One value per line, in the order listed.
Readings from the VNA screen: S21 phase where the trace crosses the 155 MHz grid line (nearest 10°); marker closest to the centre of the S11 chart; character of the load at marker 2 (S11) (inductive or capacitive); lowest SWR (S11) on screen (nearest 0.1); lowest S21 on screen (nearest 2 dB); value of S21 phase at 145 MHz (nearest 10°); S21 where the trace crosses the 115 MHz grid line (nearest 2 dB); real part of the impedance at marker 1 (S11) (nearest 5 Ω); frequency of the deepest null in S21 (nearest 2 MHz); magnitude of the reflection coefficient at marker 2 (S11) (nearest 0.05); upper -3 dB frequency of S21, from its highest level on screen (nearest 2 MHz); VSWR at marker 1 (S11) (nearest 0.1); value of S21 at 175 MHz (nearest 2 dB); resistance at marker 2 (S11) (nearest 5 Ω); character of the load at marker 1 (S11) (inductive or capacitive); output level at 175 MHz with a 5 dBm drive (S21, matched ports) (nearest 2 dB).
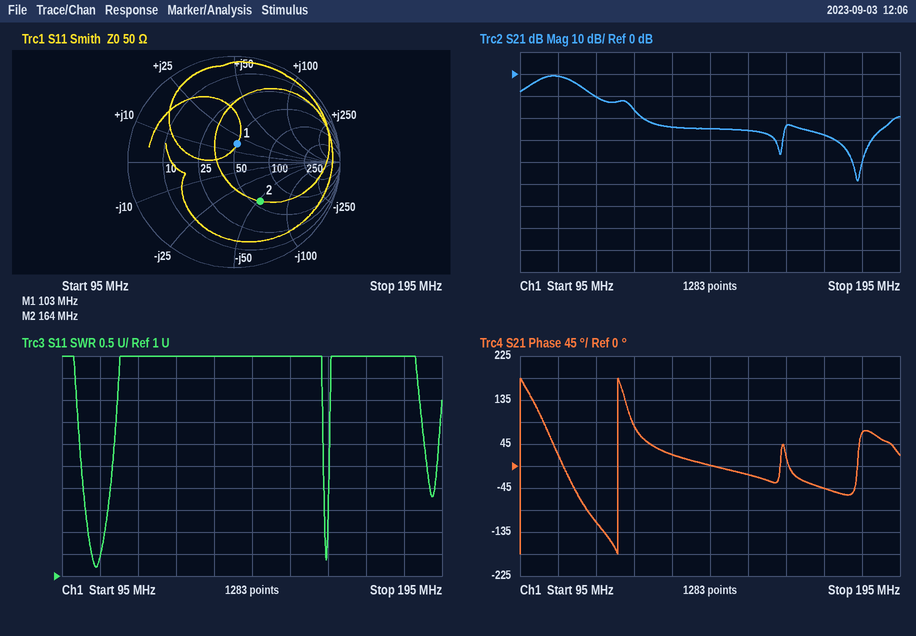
-20°
marker 1
capacitive
1.2
-48 dB
0°
-10 dB
50 Ω
184 MHz
0.45
110 MHz
1.4
-28 dB
55 Ω
inductive
-22 dBm
